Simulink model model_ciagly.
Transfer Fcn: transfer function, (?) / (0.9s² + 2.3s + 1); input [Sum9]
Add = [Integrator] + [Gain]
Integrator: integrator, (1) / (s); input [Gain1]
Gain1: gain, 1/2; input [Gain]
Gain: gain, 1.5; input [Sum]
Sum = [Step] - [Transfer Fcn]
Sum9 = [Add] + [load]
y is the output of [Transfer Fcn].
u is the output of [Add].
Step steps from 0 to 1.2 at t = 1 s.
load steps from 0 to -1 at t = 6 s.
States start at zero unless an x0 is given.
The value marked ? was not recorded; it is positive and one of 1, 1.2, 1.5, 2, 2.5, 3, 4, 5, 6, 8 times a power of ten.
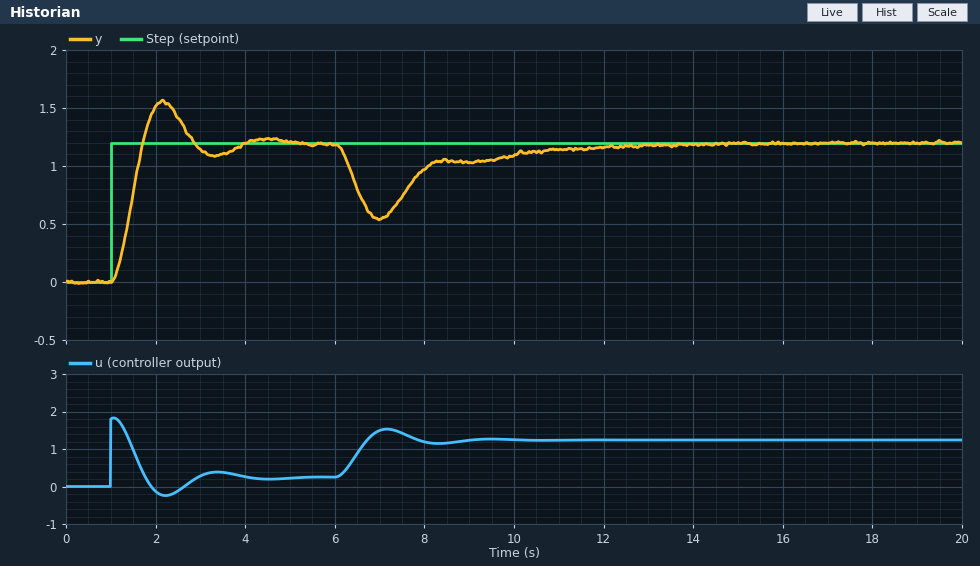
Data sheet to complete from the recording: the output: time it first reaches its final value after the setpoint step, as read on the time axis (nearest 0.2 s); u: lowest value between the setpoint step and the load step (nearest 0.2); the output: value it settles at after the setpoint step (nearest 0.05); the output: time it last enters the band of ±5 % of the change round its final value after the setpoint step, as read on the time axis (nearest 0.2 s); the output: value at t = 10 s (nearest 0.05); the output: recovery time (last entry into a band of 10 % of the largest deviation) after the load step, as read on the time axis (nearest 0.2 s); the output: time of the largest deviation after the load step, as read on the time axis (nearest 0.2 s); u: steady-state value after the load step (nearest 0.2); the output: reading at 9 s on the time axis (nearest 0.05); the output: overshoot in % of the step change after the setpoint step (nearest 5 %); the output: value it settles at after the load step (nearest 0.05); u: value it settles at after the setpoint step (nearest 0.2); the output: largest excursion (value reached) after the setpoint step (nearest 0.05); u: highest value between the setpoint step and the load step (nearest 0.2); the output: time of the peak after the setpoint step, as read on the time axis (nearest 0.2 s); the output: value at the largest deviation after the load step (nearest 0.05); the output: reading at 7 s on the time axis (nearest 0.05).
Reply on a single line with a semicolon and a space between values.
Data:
1.8 s; -0.2; 1.20; 3.8 s; 1.10; 10.8 s; 7.0 s; 1.2; 1.05; 30 %; 1.20; 0.2; 1.55; 1.8; 2.2 s; 0.55; 0.55
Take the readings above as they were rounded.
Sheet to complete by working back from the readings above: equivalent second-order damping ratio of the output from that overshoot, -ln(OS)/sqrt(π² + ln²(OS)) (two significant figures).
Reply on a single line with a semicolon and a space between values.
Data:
0.36
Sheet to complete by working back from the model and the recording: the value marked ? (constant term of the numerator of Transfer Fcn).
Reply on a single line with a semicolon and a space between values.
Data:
5
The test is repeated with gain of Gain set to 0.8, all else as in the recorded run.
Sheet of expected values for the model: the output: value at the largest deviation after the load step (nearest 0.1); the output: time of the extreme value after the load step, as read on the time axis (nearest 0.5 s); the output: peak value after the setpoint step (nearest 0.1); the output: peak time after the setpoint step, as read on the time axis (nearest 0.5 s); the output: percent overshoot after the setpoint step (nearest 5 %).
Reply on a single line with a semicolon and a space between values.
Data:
0.2; 7.5 s; 1.4; 2.5 s; 15 %
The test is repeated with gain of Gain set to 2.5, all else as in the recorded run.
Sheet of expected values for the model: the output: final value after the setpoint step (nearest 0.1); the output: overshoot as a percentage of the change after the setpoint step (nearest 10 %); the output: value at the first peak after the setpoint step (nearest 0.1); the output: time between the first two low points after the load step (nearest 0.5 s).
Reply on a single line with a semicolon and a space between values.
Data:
1.2; 40 %; 1.7; 1.5 s
